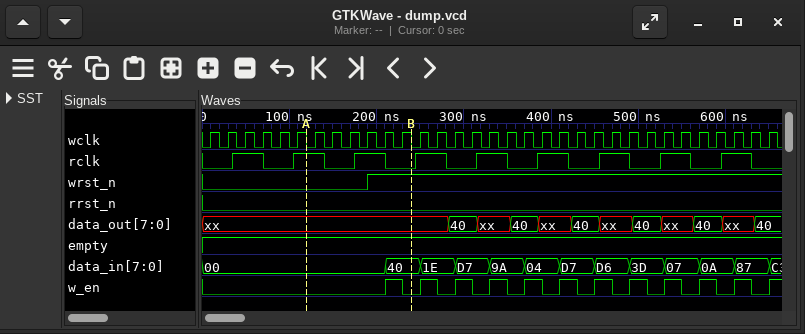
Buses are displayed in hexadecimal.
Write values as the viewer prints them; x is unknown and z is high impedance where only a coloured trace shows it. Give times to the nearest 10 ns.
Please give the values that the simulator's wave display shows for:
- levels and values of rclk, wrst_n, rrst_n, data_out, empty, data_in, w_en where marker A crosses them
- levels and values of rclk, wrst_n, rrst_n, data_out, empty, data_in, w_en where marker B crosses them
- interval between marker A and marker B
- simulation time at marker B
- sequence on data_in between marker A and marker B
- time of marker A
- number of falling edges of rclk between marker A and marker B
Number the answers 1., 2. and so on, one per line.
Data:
1. rclk=1, wrst_n=0, rrst_n=0, data_out=xx, empty=1, data_in=00, w_en=0
2. rclk=0, wrst_n=1, rrst_n=0, data_out=xx, empty=1, data_in=40, w_en=0
3. 120 ns
4. 240 ns
5. 00, 40
6. 120 ns
7. 2
